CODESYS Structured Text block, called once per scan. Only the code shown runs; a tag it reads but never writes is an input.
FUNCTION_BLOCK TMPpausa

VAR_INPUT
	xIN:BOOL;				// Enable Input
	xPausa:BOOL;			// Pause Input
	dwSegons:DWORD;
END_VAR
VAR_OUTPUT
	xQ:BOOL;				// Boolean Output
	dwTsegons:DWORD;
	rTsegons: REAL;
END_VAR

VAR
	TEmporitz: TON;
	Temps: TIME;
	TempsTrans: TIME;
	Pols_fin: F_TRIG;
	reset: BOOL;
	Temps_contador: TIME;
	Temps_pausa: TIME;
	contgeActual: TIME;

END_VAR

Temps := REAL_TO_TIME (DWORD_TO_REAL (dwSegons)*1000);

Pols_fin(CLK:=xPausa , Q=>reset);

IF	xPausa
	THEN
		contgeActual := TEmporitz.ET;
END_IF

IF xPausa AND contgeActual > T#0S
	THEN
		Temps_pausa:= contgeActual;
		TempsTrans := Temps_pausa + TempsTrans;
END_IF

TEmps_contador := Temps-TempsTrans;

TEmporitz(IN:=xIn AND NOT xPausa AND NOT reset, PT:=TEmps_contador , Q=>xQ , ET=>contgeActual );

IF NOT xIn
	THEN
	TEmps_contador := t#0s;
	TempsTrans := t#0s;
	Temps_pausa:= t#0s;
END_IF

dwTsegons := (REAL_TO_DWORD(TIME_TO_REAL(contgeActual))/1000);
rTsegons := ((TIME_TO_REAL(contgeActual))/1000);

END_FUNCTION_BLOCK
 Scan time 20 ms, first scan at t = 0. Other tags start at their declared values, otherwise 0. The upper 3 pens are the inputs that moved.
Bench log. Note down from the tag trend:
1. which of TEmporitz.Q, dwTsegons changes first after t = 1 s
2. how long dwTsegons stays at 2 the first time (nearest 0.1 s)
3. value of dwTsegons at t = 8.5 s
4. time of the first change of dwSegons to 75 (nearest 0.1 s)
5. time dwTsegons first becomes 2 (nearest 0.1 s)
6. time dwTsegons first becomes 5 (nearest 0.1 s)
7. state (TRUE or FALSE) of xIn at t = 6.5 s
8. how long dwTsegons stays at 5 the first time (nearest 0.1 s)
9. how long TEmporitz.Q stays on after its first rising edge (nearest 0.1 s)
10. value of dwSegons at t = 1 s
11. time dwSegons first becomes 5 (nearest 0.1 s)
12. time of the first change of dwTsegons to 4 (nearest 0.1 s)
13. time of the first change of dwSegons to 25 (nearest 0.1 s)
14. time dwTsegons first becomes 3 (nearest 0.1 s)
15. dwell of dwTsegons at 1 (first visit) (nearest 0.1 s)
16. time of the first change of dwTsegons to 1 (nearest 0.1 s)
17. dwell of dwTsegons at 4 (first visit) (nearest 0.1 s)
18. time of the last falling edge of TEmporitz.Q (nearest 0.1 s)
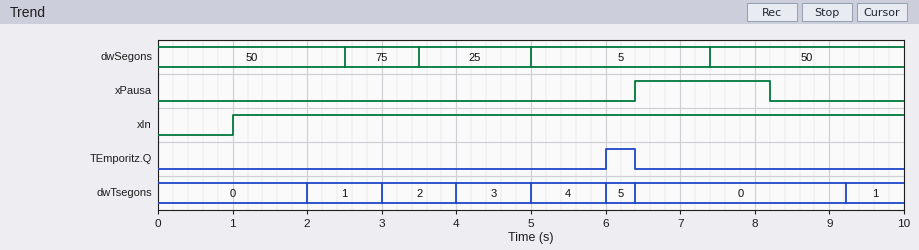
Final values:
dwTsegons
1.0 s
0
2.5 s
3.0 s
6.0 s
TRUE
0.4 s
0.4 s
50
5.0 s
5.0 s
3.5 s
4.0 s
1.0 s
2.0 s
1.0 s
6.4 s
